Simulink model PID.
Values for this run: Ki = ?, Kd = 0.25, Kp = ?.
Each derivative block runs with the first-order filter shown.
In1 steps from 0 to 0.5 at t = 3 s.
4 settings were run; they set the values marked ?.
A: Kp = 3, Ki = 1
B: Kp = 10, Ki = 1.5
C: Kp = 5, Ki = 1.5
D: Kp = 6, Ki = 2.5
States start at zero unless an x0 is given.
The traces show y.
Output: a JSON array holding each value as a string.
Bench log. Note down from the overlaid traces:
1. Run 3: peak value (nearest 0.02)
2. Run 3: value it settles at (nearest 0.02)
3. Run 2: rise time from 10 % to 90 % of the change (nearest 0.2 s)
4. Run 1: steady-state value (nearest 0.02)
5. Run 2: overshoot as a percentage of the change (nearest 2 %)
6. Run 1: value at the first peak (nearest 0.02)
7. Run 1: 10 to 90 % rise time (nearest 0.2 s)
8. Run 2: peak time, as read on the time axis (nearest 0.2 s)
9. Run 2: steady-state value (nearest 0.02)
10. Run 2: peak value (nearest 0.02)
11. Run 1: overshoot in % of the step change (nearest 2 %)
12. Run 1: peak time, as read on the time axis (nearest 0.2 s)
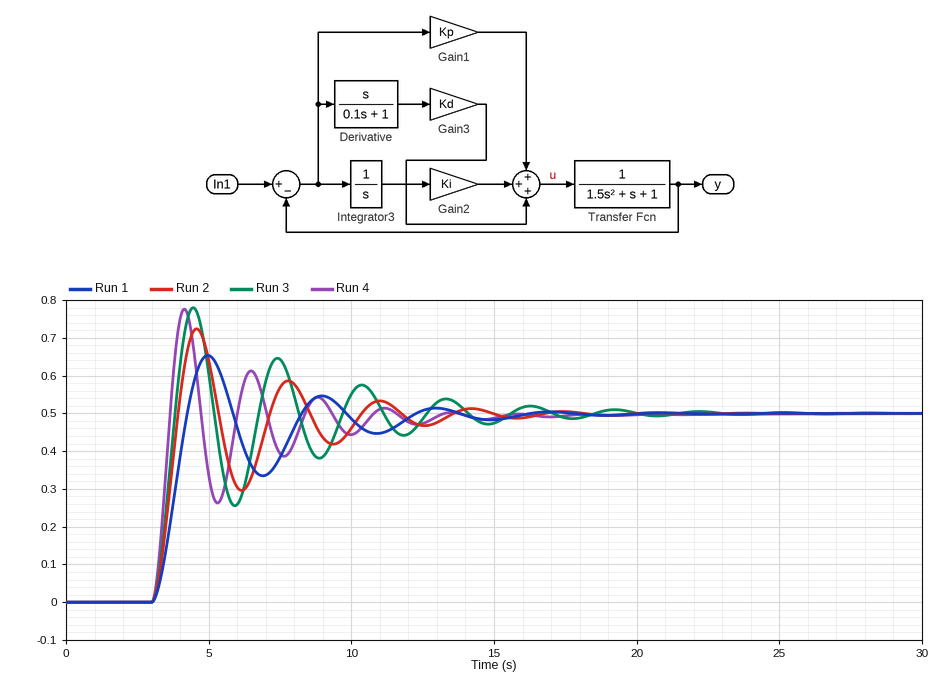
["0.78", "0.50", "0.6 s", "0.50", "44 %", "0.66", "0.8 s", "4.6 s", "0.50", "0.72", "30 %", "5.0 s"]
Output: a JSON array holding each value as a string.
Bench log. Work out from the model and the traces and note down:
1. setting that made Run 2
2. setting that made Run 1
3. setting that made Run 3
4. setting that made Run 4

["C", "A", "D", "B"]
